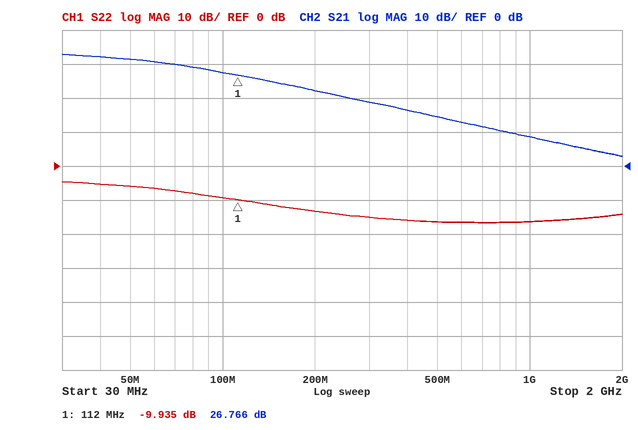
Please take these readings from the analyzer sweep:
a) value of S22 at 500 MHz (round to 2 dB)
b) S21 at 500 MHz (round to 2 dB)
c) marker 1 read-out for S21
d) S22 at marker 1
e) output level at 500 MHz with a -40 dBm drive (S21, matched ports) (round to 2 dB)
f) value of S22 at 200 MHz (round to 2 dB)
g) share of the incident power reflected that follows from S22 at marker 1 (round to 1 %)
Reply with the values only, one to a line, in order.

-16 dB
14 dB
26.766 dB
-9.935 dB
-26 dBm
-14 dB
10 %
